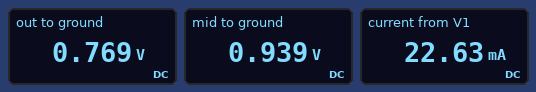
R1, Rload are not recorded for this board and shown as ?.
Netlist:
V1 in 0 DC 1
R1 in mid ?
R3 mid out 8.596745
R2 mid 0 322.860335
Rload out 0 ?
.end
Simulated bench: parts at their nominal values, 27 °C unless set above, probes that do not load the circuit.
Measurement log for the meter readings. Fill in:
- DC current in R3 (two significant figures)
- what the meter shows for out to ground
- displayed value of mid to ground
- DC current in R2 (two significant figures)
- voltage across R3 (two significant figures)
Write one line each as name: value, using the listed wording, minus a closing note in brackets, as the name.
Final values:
DC current in R3: 20 mA
what the meter shows for out to ground: 0.769 V
displayed value of mid to ground: 0.939 V
DC current in R2: 2.9 mA
voltage across R3: 170 mV
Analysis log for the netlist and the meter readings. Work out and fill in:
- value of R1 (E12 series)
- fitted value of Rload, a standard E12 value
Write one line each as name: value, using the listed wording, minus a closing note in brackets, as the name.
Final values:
value of R1: 2.7 Ω
fitted value of Rload, a standard E12 value: 39 Ω
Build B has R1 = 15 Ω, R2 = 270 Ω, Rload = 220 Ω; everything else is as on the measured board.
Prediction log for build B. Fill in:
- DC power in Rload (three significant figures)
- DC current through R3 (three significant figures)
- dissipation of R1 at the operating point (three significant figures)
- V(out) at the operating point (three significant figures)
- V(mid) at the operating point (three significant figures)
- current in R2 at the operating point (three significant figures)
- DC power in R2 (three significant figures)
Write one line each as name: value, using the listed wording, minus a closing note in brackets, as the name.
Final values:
DC power in Rload: 3.35 mW
DC current through R3: 3.90 mA
dissipation of R1 at the operating point: 779 µW
V(out) at the operating point: 858 mV
V(mid) at the operating point: 892 mV
current in R2 at the operating point: 3.30 mA
DC power in R2: 2.95 mW
